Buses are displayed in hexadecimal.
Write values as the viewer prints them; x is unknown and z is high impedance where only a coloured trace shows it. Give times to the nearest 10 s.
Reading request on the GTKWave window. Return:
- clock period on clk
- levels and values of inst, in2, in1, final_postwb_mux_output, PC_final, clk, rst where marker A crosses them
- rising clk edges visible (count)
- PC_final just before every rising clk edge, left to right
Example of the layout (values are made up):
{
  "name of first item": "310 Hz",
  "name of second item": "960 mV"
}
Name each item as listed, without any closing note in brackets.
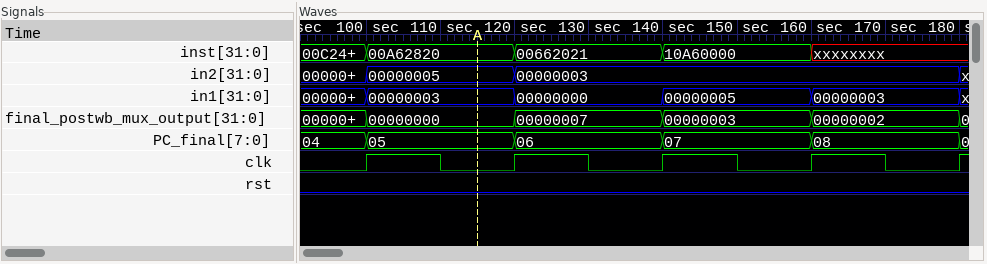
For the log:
{
  "clock period on clk": "20 s",
  "levels and values of inst, in2, in1, final_postwb_mux_output, PC_final, clk, rst where marker A crosses them": "inst=00A62820, in2=00000005, in1=00000003, final_postwb_mux_output=00000000, PC_final=05, clk=0, rst=0",
  "rising clk edges visible": "5",
  "PC_final just before every rising clk edge, left to right": "04, 05, 06, 07, 08"
}
